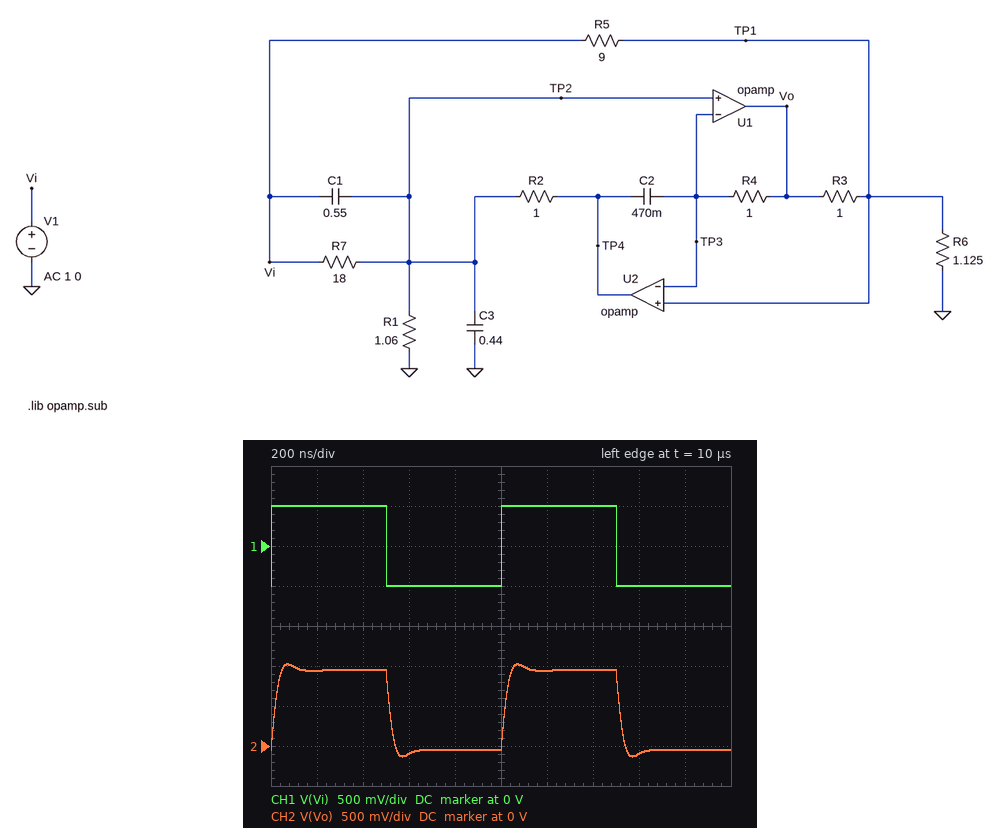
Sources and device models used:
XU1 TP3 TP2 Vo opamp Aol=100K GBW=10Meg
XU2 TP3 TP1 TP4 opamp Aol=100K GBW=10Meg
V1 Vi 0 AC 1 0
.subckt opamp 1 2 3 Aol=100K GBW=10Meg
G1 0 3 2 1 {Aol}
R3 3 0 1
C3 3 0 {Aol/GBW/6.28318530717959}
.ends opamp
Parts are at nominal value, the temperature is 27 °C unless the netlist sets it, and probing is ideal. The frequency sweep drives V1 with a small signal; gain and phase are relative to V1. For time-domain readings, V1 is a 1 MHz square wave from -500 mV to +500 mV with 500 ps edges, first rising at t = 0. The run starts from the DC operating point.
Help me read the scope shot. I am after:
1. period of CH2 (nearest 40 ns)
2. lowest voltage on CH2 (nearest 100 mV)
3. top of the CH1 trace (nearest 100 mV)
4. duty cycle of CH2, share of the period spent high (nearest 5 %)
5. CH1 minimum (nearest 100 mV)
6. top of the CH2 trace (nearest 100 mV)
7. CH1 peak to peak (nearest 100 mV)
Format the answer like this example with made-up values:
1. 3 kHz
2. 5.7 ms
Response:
1. 1.00 µs
2. -100 mV
3. 500 mV
4. 50 %
5. -500 mV
6. 1.0 V
7. 1.0 V
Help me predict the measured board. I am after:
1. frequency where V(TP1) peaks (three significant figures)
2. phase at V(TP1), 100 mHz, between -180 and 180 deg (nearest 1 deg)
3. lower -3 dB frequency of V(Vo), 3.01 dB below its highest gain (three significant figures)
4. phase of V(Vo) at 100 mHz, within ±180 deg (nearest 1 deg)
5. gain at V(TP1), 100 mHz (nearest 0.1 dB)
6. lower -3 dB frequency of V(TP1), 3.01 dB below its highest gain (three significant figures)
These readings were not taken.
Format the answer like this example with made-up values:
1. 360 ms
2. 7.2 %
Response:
1. 286 mHz
2. 41 deg
3. 203 mHz
4. 160 deg
5. -33.3 dB
6. 209 mHz
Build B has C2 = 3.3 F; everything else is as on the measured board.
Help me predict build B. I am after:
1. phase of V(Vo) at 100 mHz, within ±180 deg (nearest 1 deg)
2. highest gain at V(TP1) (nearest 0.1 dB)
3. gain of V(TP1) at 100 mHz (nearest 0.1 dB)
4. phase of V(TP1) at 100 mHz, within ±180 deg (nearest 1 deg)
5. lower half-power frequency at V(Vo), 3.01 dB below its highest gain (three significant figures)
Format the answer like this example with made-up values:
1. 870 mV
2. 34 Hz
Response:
1. 82 deg
2. -5.1 dB
3. -10.6 dB
4. 71 deg
5. 131 mHz
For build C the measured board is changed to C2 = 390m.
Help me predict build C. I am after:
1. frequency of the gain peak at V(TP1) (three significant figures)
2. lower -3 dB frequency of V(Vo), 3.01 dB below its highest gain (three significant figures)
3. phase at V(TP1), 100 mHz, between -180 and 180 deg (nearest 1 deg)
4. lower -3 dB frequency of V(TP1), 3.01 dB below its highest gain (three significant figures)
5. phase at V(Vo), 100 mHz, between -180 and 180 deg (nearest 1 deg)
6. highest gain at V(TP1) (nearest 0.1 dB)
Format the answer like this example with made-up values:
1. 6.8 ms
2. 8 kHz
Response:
1. 302 mHz
2. 223 mHz
3. 11 deg
4. 229 mHz
5. 164 deg
6. -2.0 dB
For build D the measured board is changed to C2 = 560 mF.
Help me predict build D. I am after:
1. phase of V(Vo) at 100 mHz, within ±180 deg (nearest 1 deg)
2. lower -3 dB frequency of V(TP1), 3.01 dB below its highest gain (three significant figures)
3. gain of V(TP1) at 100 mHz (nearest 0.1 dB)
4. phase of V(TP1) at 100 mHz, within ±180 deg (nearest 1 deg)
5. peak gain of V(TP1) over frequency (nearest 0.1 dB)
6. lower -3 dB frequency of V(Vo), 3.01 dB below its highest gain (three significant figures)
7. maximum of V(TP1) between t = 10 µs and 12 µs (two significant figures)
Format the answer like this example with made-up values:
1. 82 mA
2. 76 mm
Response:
1. 156 deg
2. 193 mHz
3. -31.7 dB
4. 94 deg
5. -3.2 dB
6. 187 mHz
7. 540 mV
